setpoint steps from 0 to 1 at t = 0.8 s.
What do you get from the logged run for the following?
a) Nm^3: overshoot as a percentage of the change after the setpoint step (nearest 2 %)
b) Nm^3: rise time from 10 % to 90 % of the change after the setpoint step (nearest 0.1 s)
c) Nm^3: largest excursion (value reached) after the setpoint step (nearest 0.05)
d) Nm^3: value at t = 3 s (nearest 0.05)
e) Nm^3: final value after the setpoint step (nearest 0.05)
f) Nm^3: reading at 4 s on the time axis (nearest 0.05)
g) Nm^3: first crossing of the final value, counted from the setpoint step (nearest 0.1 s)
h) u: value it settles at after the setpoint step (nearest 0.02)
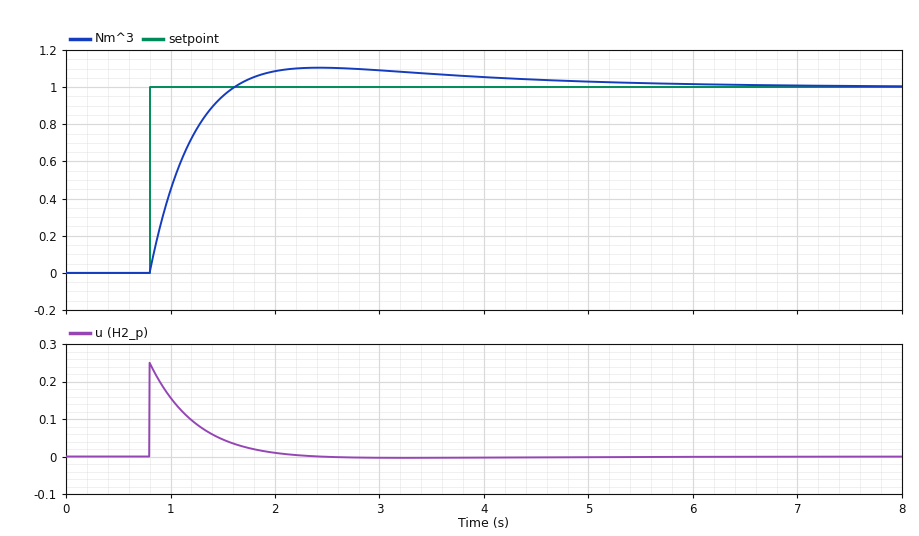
10 %
0.6 s
1.10
1.10
1.00
1.05
0.8 s
0.00
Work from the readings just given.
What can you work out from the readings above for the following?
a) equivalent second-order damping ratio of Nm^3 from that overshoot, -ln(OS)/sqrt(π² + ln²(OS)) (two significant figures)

0.59
